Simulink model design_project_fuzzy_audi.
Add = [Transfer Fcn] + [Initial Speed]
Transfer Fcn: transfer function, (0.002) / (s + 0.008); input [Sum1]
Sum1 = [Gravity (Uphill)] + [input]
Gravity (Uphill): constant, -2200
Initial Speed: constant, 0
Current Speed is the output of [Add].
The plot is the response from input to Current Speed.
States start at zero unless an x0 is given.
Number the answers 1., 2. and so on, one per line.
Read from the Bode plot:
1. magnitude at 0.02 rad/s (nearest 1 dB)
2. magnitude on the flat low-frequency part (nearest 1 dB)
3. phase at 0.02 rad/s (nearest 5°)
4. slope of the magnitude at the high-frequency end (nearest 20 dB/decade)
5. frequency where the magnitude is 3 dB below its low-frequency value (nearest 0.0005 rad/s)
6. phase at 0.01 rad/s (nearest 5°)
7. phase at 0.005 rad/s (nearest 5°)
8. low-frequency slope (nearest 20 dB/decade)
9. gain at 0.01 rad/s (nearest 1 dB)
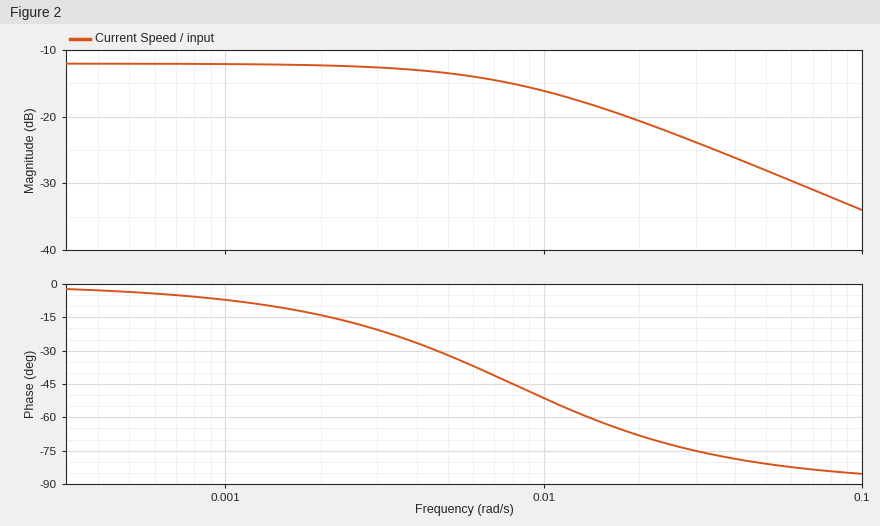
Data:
1. -21 dB
2. -12 dB
3. -70°
4. -20 dB/decade
5. 0.0080 rad/s
6. -50°
7. -30°
8. 0 dB/decade
9. -16 dB
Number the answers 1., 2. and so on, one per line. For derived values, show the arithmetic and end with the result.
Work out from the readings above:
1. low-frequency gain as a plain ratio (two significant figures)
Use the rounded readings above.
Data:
1. 10^(-12 / 20) = 0.25
